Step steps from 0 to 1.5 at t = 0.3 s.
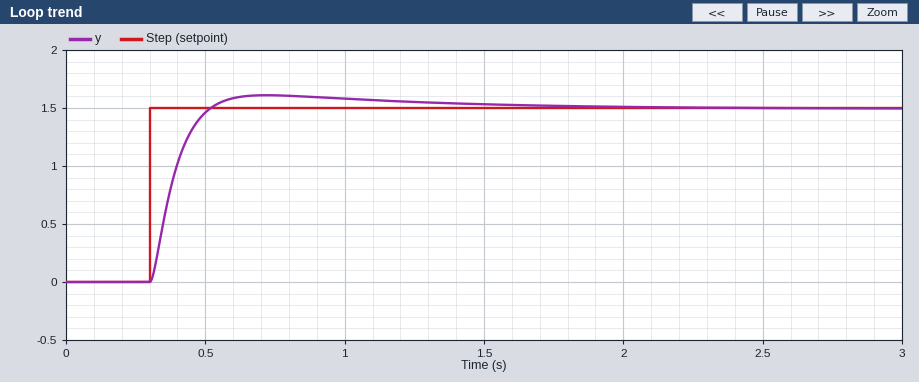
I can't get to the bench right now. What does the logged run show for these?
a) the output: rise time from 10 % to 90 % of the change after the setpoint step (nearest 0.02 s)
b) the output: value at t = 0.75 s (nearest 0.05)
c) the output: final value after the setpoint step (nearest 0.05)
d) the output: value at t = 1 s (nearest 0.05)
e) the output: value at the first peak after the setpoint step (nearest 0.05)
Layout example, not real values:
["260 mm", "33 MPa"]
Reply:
["0.14 s", "1.60", "1.50", "1.60", "1.60"]
